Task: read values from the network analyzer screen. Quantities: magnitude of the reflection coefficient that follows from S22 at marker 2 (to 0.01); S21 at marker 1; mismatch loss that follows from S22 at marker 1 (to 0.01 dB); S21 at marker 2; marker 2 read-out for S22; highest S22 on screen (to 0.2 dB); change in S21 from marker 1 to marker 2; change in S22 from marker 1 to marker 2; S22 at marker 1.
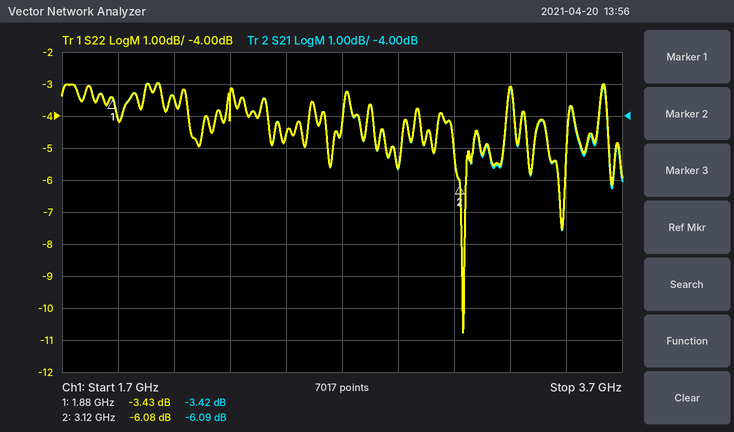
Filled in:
0.50
-3.42 dB
2.63 dB
-6.09 dB
-6.08 dB
-3.0 dB
-2.67 dB
-2.65 dB
-3.43 dB
